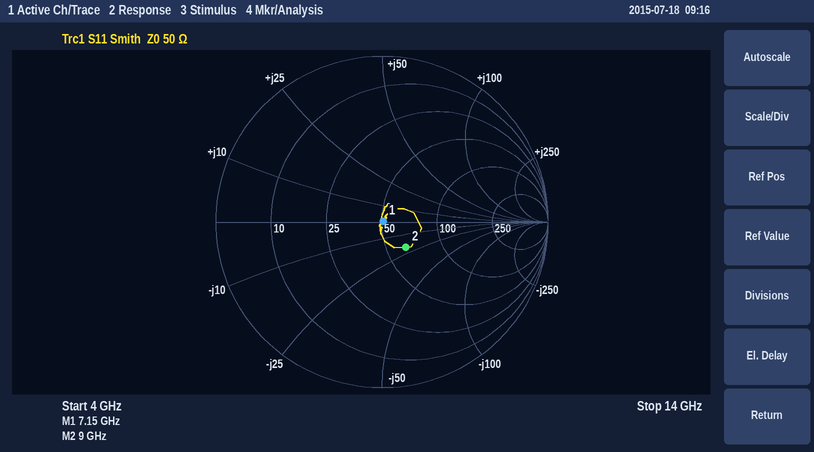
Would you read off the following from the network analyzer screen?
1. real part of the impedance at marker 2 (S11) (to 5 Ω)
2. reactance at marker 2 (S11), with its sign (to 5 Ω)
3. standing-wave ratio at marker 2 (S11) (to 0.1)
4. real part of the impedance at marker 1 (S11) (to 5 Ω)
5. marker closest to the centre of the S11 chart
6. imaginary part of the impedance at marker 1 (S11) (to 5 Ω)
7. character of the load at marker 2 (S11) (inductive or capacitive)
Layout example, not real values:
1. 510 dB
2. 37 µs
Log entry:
1. 65 Ω
2. -20 Ω
3. 1.5
4. 50 Ω
5. marker 1
6. 0 Ω
7. capacitive
